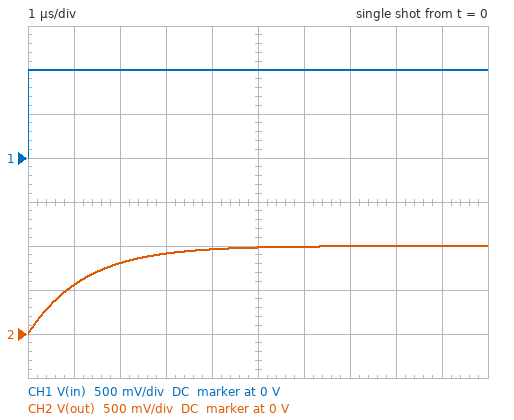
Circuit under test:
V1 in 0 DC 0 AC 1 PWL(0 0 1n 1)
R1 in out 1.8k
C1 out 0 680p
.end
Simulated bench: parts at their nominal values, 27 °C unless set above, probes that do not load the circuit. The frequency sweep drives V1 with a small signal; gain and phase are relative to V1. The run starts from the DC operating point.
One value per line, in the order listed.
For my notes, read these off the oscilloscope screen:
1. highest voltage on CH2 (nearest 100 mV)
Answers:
1.0 V
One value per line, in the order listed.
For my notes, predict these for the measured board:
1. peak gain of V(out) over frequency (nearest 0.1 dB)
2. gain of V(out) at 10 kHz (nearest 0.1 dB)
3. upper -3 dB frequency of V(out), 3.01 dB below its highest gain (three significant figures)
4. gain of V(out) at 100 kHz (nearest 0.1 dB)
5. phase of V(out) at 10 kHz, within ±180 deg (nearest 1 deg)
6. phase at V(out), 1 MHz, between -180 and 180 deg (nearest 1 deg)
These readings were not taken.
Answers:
0 dB
0 dB
130 kHz
-2.0 dB
-4 deg
-83 deg
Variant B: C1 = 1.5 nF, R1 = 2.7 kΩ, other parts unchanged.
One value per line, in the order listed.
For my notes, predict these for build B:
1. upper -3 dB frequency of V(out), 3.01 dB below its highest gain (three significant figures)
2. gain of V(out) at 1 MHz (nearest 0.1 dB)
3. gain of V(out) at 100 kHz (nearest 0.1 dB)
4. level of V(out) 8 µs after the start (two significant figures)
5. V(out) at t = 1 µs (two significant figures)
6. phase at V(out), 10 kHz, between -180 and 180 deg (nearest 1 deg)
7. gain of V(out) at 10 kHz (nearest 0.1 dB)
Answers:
39.3 kHz
-28.1 dB
-8.7 dB
860 mV
220 mV
-14 deg
-0.3 dB
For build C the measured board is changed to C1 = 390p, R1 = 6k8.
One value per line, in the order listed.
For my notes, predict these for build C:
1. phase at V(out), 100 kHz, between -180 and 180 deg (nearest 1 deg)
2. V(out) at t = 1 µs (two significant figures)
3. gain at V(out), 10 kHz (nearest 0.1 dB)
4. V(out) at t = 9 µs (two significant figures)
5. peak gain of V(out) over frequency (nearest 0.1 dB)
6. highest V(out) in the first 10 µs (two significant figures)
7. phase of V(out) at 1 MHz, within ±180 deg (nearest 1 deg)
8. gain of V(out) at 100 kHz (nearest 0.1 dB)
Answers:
-59 deg
310 mV
-0.1 dB
970 mV
0 dB
980 mV
-87 deg
-5.8 dB
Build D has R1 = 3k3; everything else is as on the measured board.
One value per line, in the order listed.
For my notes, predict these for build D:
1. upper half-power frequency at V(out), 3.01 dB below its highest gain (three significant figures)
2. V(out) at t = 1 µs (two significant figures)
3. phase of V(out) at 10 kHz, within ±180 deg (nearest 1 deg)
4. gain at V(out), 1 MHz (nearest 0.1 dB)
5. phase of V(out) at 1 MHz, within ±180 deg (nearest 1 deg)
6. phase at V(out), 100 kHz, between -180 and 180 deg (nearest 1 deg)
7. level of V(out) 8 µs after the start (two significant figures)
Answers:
70.9 kHz
360 mV
-8 deg
-23.0 dB
-86 deg
-55 deg
970 mV
